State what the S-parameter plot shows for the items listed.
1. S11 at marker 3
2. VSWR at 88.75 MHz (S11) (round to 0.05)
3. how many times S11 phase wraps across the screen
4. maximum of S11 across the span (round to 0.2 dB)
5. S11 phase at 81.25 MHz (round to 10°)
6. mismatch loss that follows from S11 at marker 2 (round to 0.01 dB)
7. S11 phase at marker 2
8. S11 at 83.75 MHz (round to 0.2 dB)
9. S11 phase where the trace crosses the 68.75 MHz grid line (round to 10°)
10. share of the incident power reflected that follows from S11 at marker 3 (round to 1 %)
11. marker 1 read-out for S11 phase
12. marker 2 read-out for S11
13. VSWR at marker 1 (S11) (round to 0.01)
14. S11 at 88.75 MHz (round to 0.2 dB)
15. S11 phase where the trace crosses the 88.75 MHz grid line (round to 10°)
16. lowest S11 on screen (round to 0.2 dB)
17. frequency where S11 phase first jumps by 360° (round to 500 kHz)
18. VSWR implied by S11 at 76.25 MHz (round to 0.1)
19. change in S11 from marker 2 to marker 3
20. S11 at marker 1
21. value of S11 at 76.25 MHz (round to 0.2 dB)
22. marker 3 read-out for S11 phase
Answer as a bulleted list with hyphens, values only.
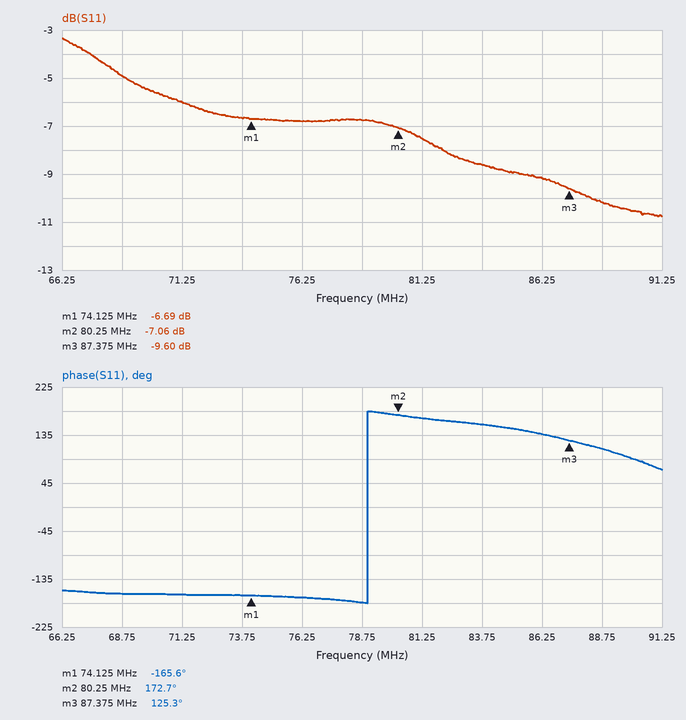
- -9.60 dB
- 1.90
- 1
- -3.4 dB
- 170°
- 0.95 dB
- 172.7°
- -8.6 dB
- -160°
- 11 %
- -165.6°
- -7.06 dB
- 2.72
- -10.2 dB
- 110°
- -10.8 dB
- 79.0 MHz
- 2.7
- -2.54 dB
- -6.69 dB
- -6.8 dB
- 125.3°
